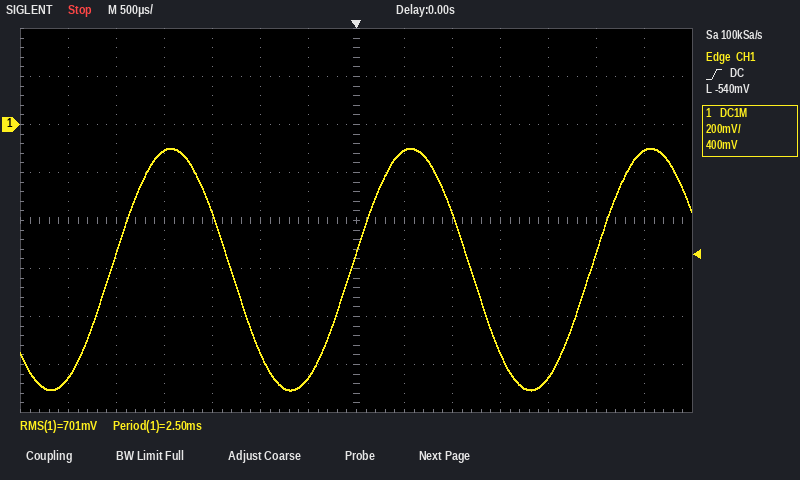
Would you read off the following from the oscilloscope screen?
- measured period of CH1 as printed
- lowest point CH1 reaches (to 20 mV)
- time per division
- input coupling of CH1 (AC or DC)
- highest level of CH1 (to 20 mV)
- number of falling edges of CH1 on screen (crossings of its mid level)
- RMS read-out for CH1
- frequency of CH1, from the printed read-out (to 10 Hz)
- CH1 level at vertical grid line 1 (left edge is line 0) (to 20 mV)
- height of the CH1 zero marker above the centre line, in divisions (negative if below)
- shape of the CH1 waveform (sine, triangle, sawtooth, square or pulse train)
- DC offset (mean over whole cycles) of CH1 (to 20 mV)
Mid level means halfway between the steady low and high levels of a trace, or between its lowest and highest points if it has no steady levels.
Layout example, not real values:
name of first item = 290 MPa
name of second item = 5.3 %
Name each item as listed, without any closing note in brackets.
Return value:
measured period of CH1 as printed = 2.50 ms
lowest point CH1 reaches = -1.10 V
time per division = 500 µs
input coupling of CH1 = DC
highest level of CH1 = -100 mV
number of falling edges of CH1 on screen = 2
RMS read-out for CH1 = 701 mV
frequency of CH1, from the printed read-out = 400 Hz
CH1 level at vertical grid line 1 (left edge is line 0) = -1.06 V
height of the CH1 zero marker above the centre line, in divisions = +2.0 div
shape of the CH1 waveform = sine
DC offset (mean over whole cycles) of CH1 = -600 mV
